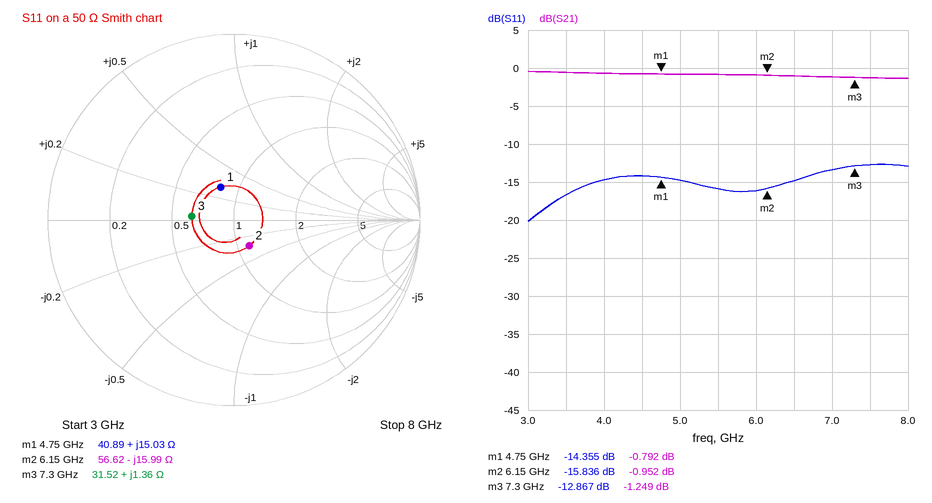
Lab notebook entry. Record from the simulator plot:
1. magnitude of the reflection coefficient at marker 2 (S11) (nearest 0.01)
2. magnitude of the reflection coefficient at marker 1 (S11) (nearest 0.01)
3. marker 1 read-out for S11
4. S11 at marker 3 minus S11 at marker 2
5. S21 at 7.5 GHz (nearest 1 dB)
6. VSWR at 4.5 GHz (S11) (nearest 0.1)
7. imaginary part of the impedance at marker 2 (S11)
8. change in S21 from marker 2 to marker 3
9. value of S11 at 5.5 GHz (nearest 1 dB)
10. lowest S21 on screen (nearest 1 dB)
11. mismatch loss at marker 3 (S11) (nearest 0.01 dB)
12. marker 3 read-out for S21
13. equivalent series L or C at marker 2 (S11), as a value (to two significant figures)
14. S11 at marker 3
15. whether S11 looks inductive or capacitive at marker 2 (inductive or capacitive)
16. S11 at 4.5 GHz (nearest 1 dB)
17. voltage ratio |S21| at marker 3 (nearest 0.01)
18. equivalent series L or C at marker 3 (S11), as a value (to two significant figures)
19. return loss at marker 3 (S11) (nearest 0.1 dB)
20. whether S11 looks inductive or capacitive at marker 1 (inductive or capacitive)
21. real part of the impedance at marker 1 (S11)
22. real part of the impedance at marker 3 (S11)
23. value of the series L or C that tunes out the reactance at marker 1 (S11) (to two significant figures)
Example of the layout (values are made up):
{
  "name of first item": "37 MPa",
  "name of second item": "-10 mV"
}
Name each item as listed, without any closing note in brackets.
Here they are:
{
  "magnitude of the reflection coefficient at marker 2 (S11)": "0.16",
  "magnitude of the reflection coefficient at marker 1 (S11)": "0.19",
  "marker 1 read-out for S11": "-14.355 dB",
  "S11 at marker 3 minus S11 at marker 2": "2.969 dB",
  "S21 at 7.5 GHz": "-1 dB",
  "VSWR at 4.5 GHz (S11)": "1.5",
  "imaginary part of the impedance at marker 2": "-15.99 Ω",
  "change in S21 from marker 2 to marker 3": "-0.297 dB",
  "value of S11 at 5.5 GHz": "-16 dB",
  "lowest S21 on screen": "-1 dB",
  "mismatch loss at marker 3 (S11)": "0.23 dB",
  "marker 3 read-out for S21": "-1.249 dB",
  "equivalent series L or C at marker 2 (S11), as a value": "1.6 pF",
  "S11 at marker 3": "-12.867 dB",
  "whether S11 looks inductive or capacitive at marker 2": "capacitive",
  "S11 at 4.5 GHz": "-14 dB",
  "voltage ratio |S21| at marker 3": "0.87",
  "equivalent series L or C at marker 3 (S11), as a value": "30 pH",
  "return loss at marker 3 (S11)": "12.9 dB",
  "whether S11 looks inductive or capacitive at marker 1": "inductive",
  "real part of the impedance at marker 1": "40.89 Ω",
  "real part of the impedance at marker 3": "31.52 Ω",
  "value of the series L or C that tunes out the reactance at marker 1 (S11)": "2.2 pF"
}
